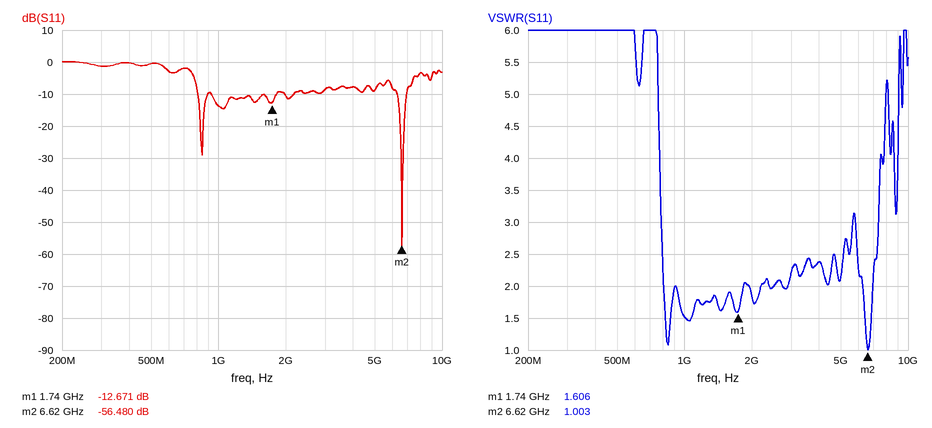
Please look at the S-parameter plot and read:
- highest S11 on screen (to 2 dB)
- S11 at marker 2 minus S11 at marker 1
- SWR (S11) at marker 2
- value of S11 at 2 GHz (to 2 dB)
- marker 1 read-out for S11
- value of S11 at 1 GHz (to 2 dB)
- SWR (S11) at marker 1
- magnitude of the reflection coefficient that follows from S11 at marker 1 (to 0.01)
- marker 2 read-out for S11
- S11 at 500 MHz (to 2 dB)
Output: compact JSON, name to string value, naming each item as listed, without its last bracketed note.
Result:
{"highest S11 on screen": "0 dB", "S11 at marker 2 minus S11 at marker 1": "-43.809 dB", "SWR (S11) at marker 2": "1.003", "value of S11 at 2 GHz": "-10 dB", "marker 1 read-out for S11": "-12.671 dB", "value of S11 at 1 GHz": "-14 dB", "SWR (S11) at marker 1": "1.606", "magnitude of the reflection coefficient that follows from S11 at marker 1": "0.23", "marker 2 read-out for S11": "-56.480 dB", "S11 at 500 MHz": "0 dB"}
